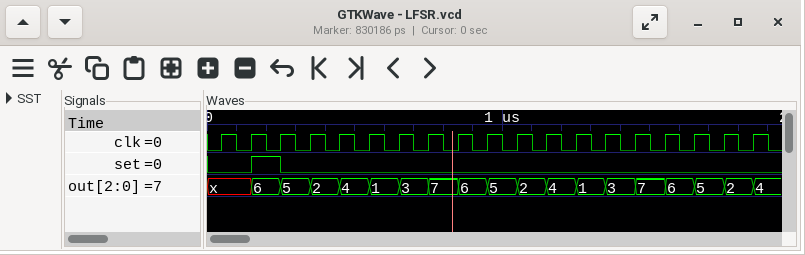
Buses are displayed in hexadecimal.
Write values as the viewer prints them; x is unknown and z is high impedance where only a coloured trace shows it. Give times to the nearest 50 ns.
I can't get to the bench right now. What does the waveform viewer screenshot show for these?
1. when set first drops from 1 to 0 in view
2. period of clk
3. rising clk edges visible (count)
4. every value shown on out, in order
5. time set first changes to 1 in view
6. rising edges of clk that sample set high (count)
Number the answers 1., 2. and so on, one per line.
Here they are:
1. 250 ns
2. 100 ns
3. 19
4. x, 6, 5, 2, 4, 1, 3, 7, 6, 5, 2, 4, 1, 3, 7, 6, 5, 2, 4
5. 150 ns
6. 1
